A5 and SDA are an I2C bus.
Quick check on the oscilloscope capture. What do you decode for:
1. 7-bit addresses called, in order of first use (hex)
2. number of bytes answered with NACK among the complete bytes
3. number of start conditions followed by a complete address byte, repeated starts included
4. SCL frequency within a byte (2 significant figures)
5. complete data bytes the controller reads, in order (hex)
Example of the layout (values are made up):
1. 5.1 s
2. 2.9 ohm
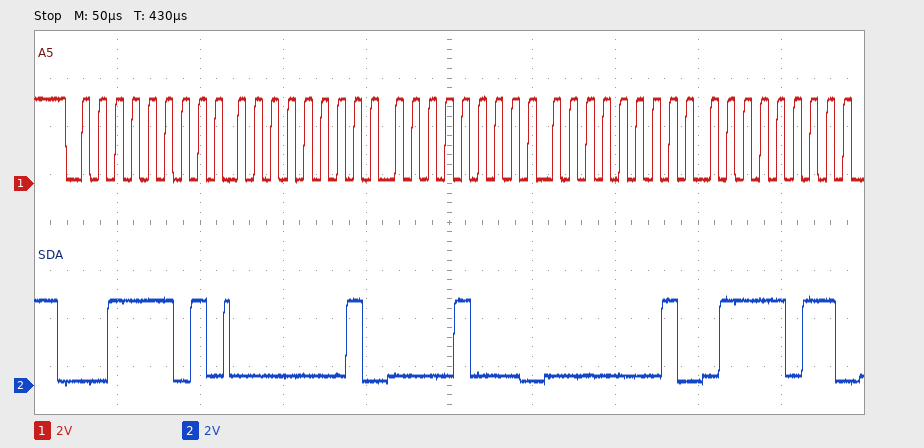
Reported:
1. 0x1E
2. 0
3. 1
4. 100 kHz
5. 01 08 01 7B
